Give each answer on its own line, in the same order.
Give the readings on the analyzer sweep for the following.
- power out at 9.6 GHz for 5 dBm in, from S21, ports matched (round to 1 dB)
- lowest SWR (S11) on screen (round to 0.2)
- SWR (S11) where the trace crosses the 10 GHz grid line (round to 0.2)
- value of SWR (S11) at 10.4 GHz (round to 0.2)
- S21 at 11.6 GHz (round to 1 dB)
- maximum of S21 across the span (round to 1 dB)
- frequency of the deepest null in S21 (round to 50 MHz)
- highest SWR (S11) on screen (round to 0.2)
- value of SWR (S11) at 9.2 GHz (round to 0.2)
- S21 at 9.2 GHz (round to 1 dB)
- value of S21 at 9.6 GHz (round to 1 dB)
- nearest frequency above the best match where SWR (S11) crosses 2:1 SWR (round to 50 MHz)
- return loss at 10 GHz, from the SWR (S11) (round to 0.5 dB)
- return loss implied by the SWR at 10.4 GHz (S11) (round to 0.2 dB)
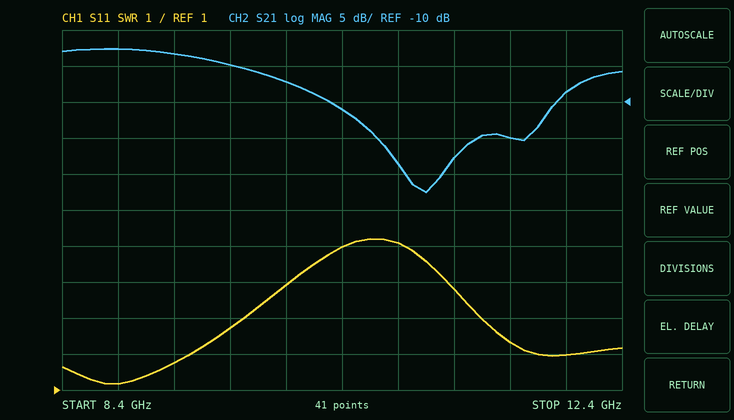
0 dBm
1.2
4.0
5.0
-15 dB
-3 dB
11.00 GHz
5.2
1.8
-3 dB
-5 dB
9.30 GHz
4.5 dB
3.6 dB
